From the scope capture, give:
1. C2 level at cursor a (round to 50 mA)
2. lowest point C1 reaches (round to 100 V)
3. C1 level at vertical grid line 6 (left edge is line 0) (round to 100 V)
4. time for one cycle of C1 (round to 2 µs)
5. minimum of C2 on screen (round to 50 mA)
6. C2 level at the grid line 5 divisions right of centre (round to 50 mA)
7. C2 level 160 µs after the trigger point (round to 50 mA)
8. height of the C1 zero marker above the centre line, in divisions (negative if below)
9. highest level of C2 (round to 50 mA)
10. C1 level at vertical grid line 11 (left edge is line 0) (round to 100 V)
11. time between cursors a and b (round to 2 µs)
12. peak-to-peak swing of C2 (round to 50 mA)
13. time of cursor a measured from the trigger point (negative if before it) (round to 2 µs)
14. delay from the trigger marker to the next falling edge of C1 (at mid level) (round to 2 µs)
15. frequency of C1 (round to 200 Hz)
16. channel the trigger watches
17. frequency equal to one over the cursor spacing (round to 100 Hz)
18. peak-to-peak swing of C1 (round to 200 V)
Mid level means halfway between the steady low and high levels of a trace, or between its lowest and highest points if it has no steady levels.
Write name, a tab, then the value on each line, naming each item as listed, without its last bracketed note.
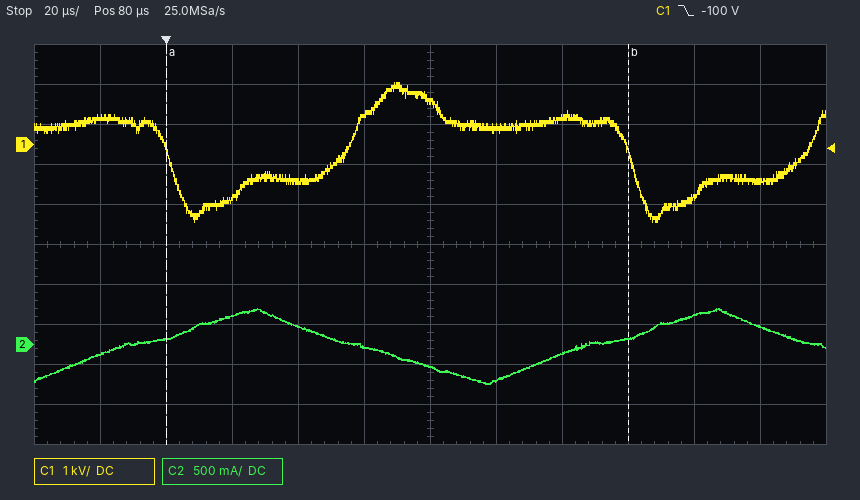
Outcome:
C2 level at cursor a	50 mA
lowest point C1 reaches	-2.0 kV
C1 level at vertical grid line 6 (left edge is line 0)	1.1 kV
time for one cycle of C1	140 µs
minimum of C2 on screen	-500 mA
C2 level at the grid line 5 divisions right of centre	200 mA
C2 level 160 µs after the trigger point	350 mA
height of the C1 zero marker above the centre line, in divisions	+2.5 div
highest level of C2	450 mA
C1 level at vertical grid line 11 (left edge is line 0)	-900 V
time between cursors a and b	140 µs
peak-to-peak swing of C2	950 mA
time of cursor a measured from the trigger point (negative if before it)	0 µs
delay from the trigger marker to the next falling edge of C1 (at mid level)	140 µs
frequency of C1	7.2 kHz
channel the trigger watches	C1
frequency equal to one over the cursor spacing	7.1 kHz
peak-to-peak swing of C1	3.6 kV
